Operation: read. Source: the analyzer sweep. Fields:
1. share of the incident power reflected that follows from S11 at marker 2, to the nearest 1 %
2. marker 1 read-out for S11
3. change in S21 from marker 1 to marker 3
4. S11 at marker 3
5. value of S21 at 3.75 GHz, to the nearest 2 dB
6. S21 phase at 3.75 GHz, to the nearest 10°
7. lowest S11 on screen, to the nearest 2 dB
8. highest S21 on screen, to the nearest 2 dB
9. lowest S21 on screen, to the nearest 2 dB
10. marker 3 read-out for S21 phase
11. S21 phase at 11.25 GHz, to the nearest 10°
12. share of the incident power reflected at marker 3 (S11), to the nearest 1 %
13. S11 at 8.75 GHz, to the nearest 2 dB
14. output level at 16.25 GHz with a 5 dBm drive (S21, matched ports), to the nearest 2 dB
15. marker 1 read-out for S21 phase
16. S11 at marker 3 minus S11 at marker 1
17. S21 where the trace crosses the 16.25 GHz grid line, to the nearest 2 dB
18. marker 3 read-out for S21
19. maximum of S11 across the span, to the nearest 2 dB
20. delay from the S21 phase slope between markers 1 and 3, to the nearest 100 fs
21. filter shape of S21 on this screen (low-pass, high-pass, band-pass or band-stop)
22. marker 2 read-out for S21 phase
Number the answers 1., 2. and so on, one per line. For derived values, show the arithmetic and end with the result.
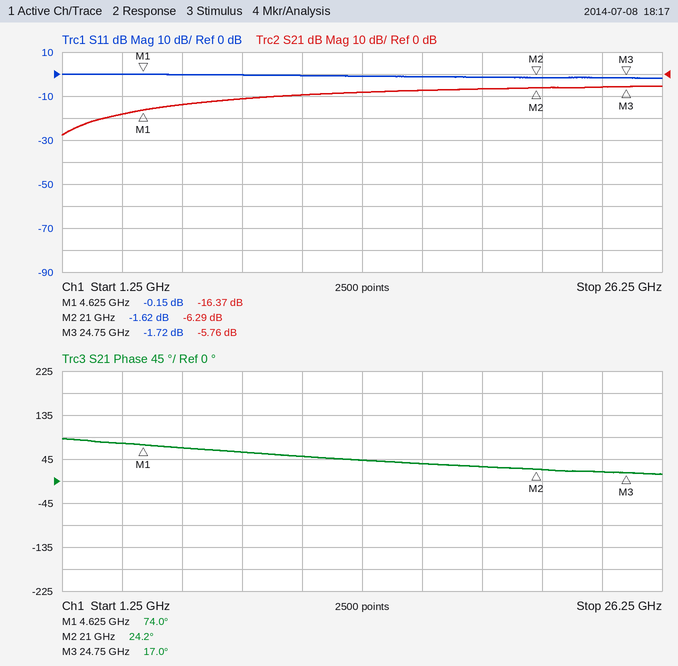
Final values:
1. 10^(-1.62/10) ≈ 69 %
2. -0.15 dB
3. -5.76 − (-16.37) = 10.61 dB
4. -1.72 dB
5. -18 dB
6. 80°
7. -2 dB
8. -6 dB
9. -28 dB
10. 17.0°
11. 50°
12. 10^(-1.72/10) ≈ 67 %
13. 0 dB
14. 5 dBm + (-8 dB) = -2 dBm
15. 74.0°
16. -1.72 − (-0.15) = -1.57 dB
17. -8 dB
18. -5.76 dB
19. 0 dB
20. −(17° − (74°))/(360° × 20.125 GHz) ≈ 7.9 ps
21. high-pass
22. 24.2°
